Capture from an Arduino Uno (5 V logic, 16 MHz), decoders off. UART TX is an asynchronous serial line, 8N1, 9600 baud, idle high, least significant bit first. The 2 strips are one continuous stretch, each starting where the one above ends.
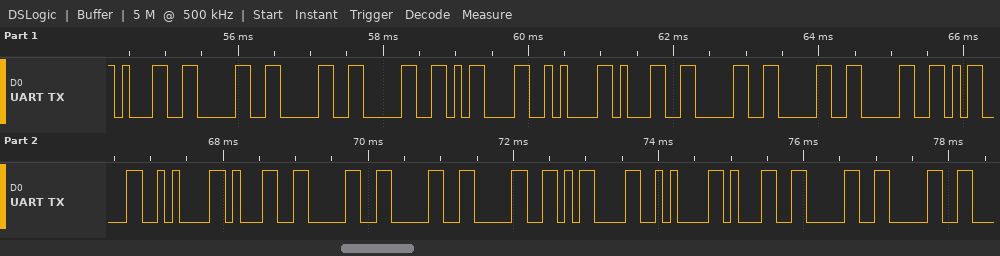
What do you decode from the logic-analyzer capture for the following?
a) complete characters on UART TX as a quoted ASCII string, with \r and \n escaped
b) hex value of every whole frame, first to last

"1000\r\n1000\r\n1000\r\n100"
31 30 30 30 0D 0A 31 30 30 30 0D 0A 31 30 30 30 0D 0A 31 30 30
